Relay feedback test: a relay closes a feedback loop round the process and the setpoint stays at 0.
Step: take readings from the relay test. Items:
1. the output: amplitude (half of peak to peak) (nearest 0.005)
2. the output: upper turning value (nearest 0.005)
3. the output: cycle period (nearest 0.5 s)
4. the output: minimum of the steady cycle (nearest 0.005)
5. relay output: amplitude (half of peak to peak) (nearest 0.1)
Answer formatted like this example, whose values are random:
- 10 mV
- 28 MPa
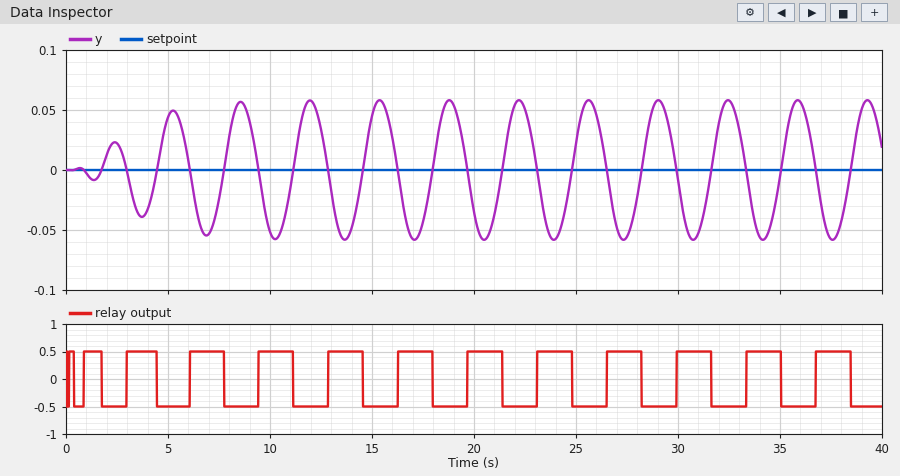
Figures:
- 0.060
- 0.060
- 3.5 s
- -0.060
- 0.5
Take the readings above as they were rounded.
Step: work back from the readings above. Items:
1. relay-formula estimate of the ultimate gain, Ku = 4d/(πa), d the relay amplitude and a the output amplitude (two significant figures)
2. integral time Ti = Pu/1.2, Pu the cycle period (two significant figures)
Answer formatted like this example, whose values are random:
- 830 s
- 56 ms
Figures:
- 11
- 2.9 s
